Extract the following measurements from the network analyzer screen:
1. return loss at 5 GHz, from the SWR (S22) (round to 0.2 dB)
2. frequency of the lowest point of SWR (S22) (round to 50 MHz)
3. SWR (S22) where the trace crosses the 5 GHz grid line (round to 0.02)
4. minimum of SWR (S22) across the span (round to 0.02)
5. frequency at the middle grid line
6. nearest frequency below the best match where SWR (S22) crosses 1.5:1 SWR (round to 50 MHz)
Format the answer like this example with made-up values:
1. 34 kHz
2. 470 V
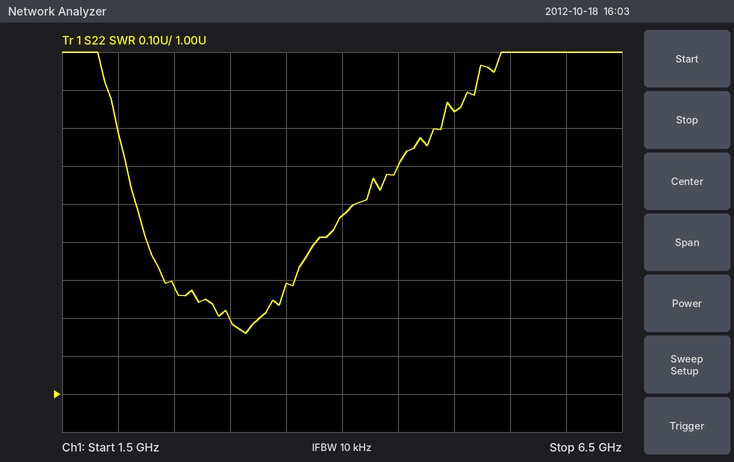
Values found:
1. 11.4 dB
2. 3.15 GHz
3. 1.74
4. 1.16
5. 4 GHz
6. 2.15 GHz
